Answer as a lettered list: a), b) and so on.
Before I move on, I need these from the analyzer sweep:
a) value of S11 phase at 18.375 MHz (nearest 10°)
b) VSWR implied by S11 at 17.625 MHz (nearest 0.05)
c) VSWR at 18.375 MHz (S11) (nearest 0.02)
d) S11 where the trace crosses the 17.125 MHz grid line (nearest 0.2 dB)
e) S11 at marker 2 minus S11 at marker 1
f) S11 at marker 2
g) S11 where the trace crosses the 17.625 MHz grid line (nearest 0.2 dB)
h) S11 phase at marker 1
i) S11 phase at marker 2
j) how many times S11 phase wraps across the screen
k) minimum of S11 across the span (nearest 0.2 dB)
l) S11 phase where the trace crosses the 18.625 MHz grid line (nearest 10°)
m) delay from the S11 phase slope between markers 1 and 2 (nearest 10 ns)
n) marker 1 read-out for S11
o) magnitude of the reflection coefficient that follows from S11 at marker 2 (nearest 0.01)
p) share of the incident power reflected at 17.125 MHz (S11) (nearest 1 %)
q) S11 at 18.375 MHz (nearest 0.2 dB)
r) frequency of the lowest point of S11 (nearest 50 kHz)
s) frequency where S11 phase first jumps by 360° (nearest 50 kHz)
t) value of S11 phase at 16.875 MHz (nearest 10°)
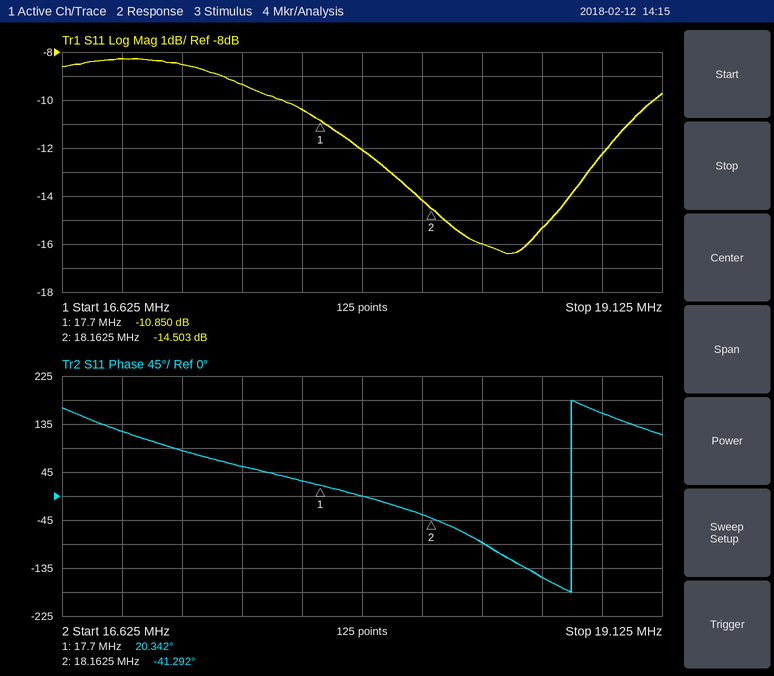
a) -90°
b) 1.85
c) 1.38
d) -8.6 dB
e) -3.653 dB
f) -14.503 dB
g) -10.4 dB
h) 20.342°
i) -41.292°
j) 1
k) -16.4 dB
l) -150°
m) 370 ns
n) -10.850 dB
o) 0.19
p) 14 %
q) -16.0 dB
r) 18.50 MHz
s) 18.75 MHz
t) 120°
